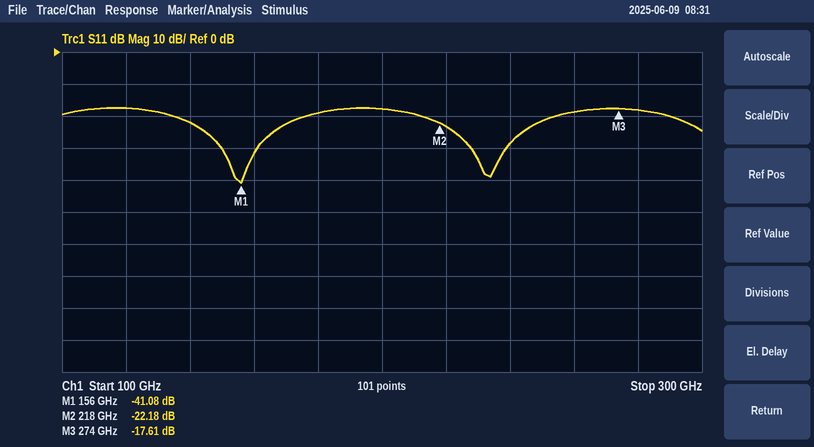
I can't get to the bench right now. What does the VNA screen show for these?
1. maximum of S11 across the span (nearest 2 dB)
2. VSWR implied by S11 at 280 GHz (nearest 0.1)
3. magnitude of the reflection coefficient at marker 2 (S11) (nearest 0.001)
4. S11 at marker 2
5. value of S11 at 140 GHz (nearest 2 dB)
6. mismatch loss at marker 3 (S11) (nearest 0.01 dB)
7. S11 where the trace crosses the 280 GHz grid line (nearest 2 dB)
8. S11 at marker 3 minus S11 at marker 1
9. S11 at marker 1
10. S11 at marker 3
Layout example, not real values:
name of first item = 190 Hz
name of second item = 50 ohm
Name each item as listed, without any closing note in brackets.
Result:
maximum of S11 across the span = -18 dB
VSWR implied by S11 at 280 GHz = 1.3
magnitude of the reflection coefficient at marker 2 (S11) = 0.078
S11 at marker 2 = -22.18 dB
value of S11 at 140 GHz = -22 dB
mismatch loss at marker 3 (S11) = 0.08 dB
S11 where the trace crosses the 280 GHz grid line = -18 dB
S11 at marker 3 minus S11 at marker 1 = 23.47 dB
S11 at marker 1 = -41.08 dB
S11 at marker 3 = -17.61 dB
